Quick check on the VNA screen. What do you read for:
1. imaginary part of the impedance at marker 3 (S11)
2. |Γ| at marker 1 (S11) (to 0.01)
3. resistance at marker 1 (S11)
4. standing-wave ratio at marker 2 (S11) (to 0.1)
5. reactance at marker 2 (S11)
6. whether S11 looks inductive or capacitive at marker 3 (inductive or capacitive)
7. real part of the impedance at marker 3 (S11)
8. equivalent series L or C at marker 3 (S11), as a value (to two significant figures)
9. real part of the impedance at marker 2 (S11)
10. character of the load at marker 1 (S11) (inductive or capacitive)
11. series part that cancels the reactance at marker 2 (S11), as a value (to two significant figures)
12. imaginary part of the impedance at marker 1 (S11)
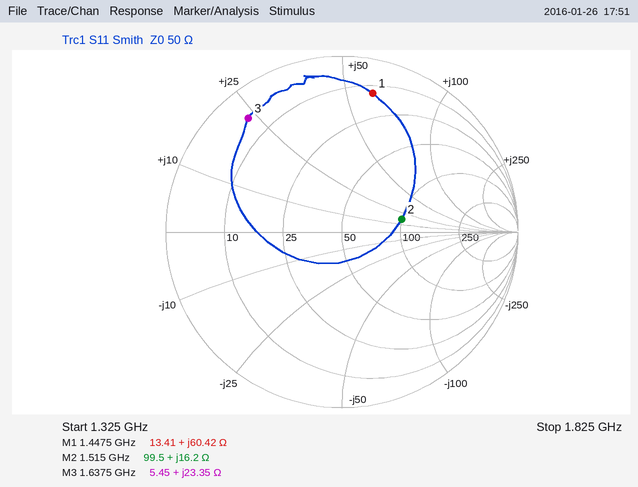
+23.35 Ω
0.81
13.41 Ω
2.1
+16.2 Ω
inductive
5.45 Ω
2.3 nH
99.5 Ω
inductive
6.5 pF
+60.42 Ω
